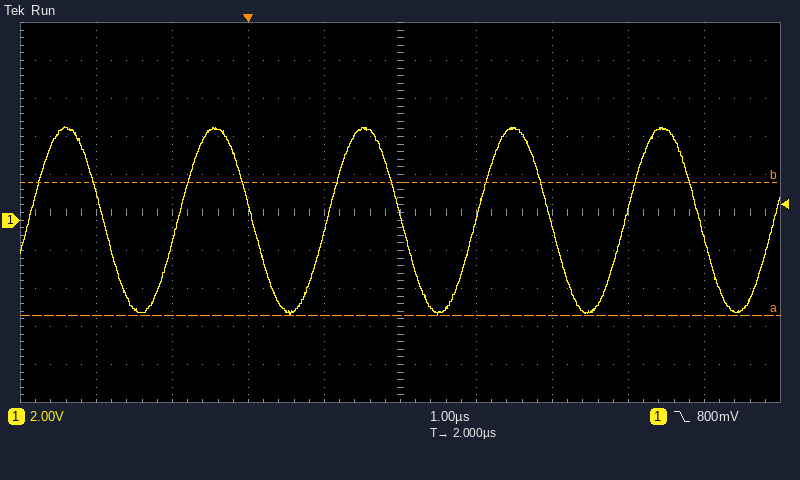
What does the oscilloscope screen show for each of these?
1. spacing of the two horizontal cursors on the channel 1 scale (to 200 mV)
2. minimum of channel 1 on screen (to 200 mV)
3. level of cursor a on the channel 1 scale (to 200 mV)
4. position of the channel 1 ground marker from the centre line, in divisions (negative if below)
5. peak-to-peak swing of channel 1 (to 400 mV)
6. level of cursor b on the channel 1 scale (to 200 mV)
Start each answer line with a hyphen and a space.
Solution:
- 7.0 V
- -5.0 V
- -5.0 V
- -0.2 div
- 10.0 V
- 2.0 V
